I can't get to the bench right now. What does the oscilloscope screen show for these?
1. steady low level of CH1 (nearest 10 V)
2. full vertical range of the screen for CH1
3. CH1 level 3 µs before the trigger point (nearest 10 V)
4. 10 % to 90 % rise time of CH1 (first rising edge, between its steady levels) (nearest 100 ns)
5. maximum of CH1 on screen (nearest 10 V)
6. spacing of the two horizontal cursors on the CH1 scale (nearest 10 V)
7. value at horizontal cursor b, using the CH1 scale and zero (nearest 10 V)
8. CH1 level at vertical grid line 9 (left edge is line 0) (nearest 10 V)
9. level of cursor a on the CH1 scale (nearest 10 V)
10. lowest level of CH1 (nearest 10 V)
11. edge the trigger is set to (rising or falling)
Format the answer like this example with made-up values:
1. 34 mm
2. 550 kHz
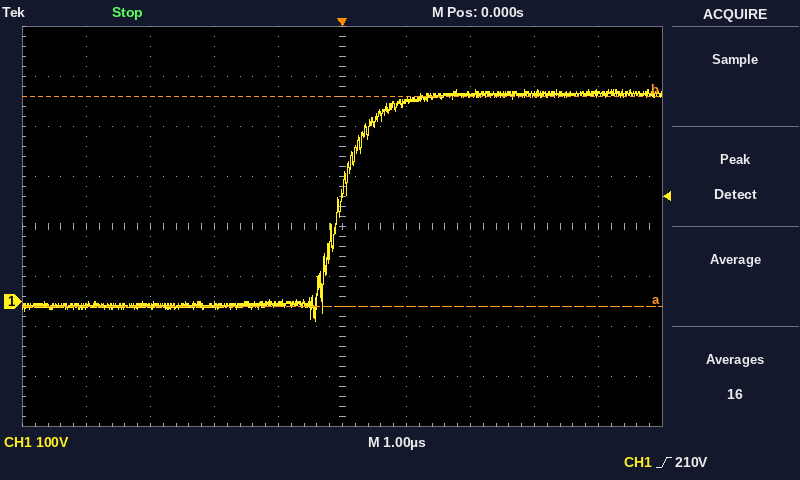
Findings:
1. -10 V
2. 800 V
3. -10 V
4. 900 ns
5. 420 V
6. 420 V
7. 410 V
8. 420 V
9. -10 V
10. -40 V
11. rising
